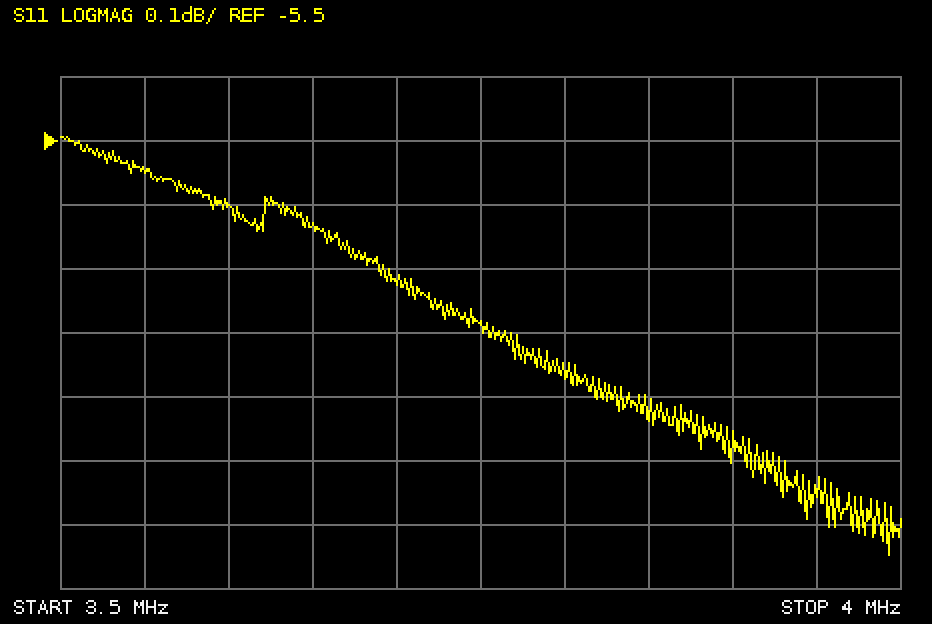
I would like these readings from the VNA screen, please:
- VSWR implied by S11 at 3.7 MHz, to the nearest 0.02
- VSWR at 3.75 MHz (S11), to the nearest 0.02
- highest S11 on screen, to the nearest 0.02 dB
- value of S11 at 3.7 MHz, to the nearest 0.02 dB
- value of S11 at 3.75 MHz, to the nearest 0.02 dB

3.14
3.12
-5.50 dB
-5.72 dB
-5.78 dB
